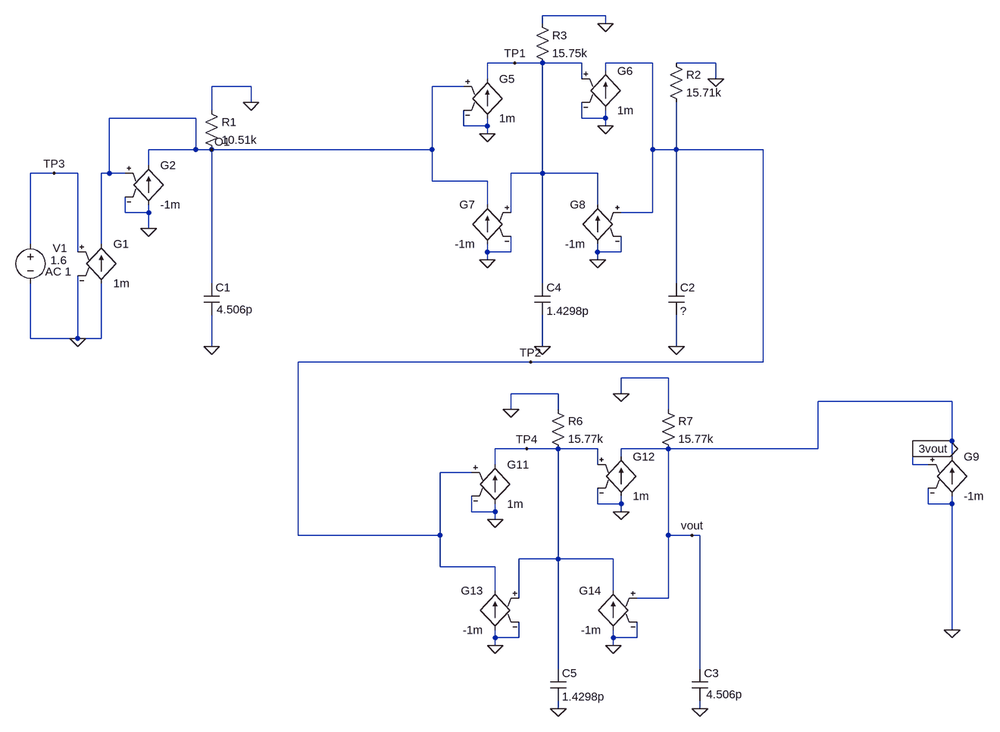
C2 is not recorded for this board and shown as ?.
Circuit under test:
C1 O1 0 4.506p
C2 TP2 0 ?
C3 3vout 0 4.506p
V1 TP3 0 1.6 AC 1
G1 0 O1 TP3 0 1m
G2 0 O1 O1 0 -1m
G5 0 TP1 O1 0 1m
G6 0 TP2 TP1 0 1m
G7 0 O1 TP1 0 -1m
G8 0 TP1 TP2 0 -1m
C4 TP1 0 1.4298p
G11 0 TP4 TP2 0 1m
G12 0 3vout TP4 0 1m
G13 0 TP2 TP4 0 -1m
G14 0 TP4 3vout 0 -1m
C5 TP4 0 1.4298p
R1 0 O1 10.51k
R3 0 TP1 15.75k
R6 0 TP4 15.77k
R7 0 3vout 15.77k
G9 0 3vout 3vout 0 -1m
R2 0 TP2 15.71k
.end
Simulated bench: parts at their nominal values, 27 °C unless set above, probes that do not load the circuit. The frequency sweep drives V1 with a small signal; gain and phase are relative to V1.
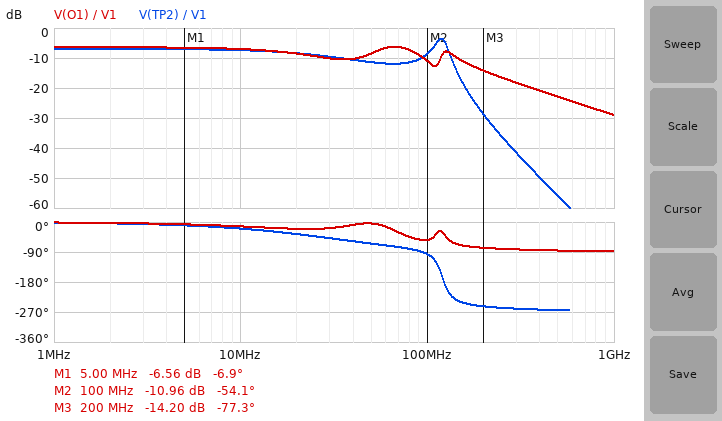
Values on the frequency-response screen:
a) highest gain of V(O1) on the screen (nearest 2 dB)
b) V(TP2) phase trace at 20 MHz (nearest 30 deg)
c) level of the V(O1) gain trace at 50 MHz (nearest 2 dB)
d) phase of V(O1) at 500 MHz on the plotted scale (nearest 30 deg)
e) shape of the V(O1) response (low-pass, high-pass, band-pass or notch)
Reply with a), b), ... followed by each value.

a) -6 dB
b) -30 deg
c) -8 dB
d) -90 deg
e) low-pass
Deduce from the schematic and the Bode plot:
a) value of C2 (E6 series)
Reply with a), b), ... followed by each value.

a) 3.3 pF
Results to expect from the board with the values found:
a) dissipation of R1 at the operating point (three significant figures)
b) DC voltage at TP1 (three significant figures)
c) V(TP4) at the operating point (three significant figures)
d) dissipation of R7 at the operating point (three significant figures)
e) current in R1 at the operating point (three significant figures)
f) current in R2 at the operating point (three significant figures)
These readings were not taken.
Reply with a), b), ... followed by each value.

a) 55.9 µW
b) 761 mV
c) 715 mV
d) 28.7 µW
e) 72.9 µA
f) 45.7 µA
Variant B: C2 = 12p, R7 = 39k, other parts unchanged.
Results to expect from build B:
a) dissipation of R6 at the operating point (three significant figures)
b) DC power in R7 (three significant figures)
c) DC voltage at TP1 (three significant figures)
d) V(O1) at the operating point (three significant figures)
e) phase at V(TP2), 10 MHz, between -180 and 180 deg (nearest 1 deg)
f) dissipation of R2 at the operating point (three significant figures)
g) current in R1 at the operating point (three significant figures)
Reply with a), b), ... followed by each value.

a) 31.3 µW
b) 12.0 µW
c) 749 mV
d) 777 mV
e) -33 deg
f) 33.9 µW
g) 73.9 µA
